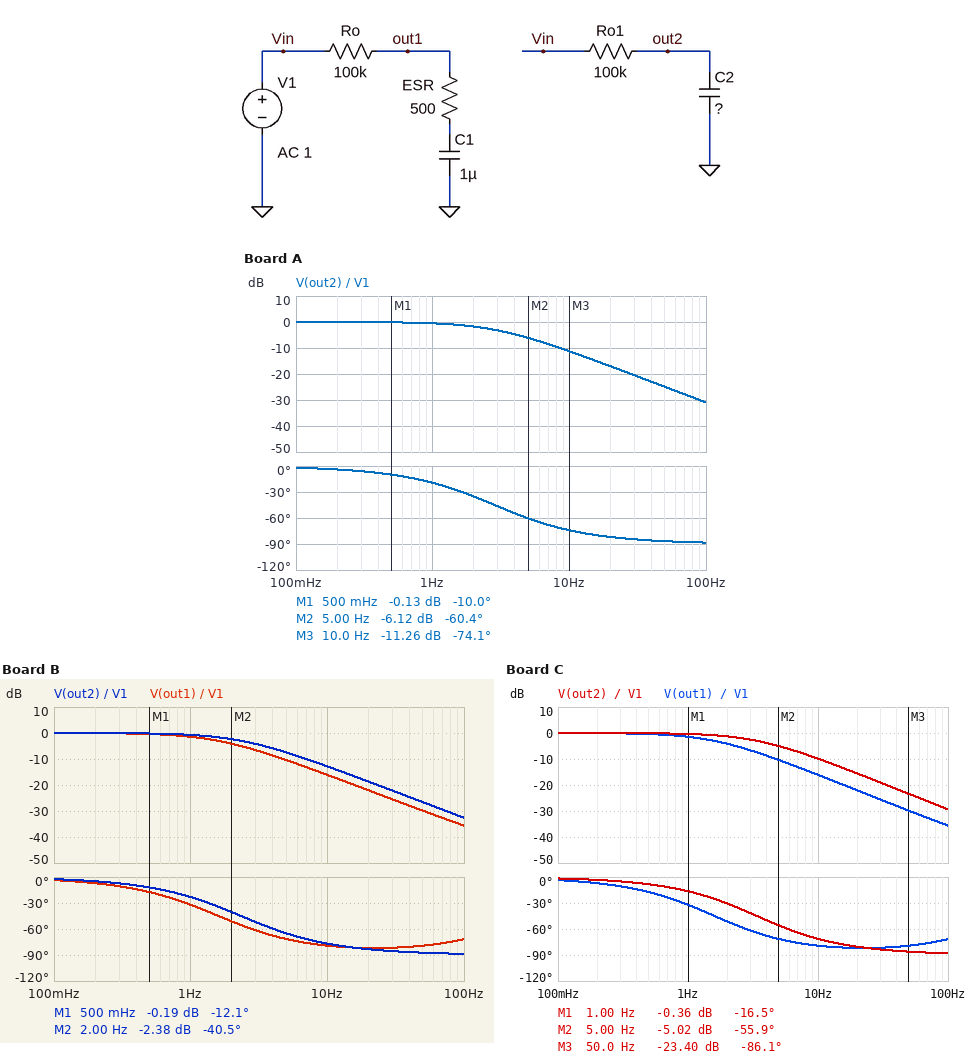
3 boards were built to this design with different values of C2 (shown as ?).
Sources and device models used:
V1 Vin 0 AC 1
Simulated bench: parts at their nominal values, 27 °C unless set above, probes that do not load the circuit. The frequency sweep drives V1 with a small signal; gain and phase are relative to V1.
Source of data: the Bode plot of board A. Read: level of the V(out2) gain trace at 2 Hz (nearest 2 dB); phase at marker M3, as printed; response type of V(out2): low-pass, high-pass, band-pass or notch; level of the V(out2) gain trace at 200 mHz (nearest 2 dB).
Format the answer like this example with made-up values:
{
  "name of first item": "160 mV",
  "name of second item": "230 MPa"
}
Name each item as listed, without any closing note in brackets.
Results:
{
  "level of the V(out2) gain trace at 2 Hz": "-2 dB",
  "phase at marker M3, as printed": "-74.1 deg",
  "response type of V(out2): low-pass, high-pass, band-pass or notch": "low-pass",
  "level of the V(out2) gain trace at 200 mHz": "0 dB"
}
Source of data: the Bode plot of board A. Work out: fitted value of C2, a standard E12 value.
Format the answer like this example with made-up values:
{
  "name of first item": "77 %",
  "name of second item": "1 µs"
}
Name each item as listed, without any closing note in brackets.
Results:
{
  "fitted value of C2, a standard E12 value": "560 nF"
}
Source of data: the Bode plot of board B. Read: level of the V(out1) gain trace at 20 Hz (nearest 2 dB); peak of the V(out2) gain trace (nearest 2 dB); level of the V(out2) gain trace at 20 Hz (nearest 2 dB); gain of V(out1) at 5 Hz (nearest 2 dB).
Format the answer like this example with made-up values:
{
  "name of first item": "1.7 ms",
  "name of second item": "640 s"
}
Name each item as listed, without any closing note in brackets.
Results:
{
  "level of the V(out1) gain trace at 20 Hz": "-22 dB",
  "peak of the V(out2) gain trace": "0 dB",
  "level of the V(out2) gain trace at 20 Hz": "-18 dB",
  "gain of V(out1) at 5 Hz": "-10 dB"
}
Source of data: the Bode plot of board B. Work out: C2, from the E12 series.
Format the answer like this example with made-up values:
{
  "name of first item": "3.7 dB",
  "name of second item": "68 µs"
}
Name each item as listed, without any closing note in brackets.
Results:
{
  "C2, from the E12 series": "680 nF"
}
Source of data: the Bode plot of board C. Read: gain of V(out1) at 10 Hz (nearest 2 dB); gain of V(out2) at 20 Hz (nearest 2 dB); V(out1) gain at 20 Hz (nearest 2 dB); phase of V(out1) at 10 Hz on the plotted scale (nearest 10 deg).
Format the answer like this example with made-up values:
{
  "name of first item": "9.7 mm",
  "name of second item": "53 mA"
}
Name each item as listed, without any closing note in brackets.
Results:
{
  "gain of V(out1) at 10 Hz": "-16 dB",
  "gain of V(out2) at 20 Hz": "-16 dB",
  "V(out1) gain at 20 Hz": "-22 dB",
  "phase of V(out1) at 10 Hz on the plotted scale": "-80 deg"
}
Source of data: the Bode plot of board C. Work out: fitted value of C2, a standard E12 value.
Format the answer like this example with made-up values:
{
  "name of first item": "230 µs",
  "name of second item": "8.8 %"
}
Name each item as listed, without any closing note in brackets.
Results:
{
  "fitted value of C2, a standard E12 value": "470 nF"
}
